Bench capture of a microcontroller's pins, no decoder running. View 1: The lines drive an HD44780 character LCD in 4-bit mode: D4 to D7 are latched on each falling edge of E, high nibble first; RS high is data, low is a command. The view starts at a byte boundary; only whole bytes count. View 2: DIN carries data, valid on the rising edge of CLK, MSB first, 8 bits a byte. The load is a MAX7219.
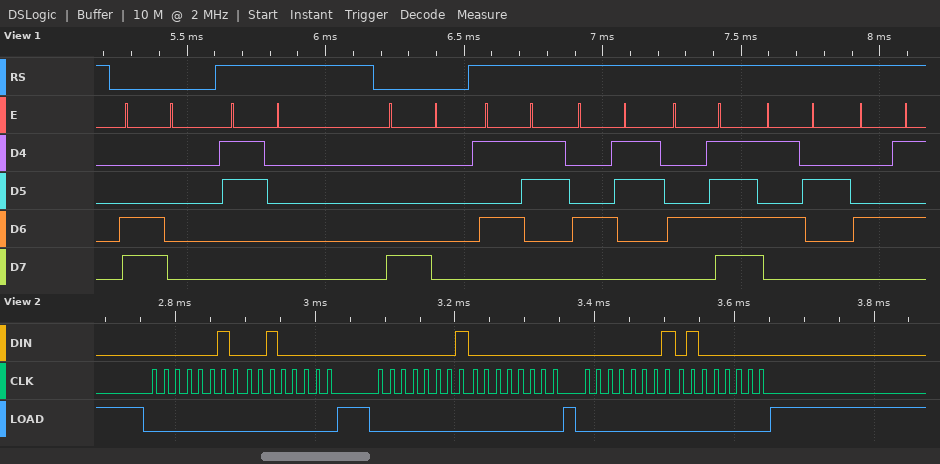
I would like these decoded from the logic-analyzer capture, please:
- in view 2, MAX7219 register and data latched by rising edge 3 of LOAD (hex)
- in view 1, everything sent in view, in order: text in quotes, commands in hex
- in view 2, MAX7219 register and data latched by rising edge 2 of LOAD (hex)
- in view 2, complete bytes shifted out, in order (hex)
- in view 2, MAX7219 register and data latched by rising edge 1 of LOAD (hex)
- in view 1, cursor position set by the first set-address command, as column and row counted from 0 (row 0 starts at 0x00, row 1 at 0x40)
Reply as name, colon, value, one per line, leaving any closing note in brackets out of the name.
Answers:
in view 2, MAX7219 register and data latched by rising edge 3 of LOAD: register 0x1, data 0x40
in view 1, everything sent in view, in order: text in quotes, commands in hex: 0xC0 "0" 0x80 "SCORE"
in view 2, MAX7219 register and data latched by rising edge 2 of LOAD: register 0x1, data 0x00
in view 2, complete bytes shifted out, in order: 0x02 0x20 0x01 0x00 0x01 0x40
in view 2, MAX7219 register and data latched by rising edge 1 of LOAD: register 0x2, data 0x20
in view 1, cursor position set by the first set-address command, as column and row counted from 0: column 0, row 1
